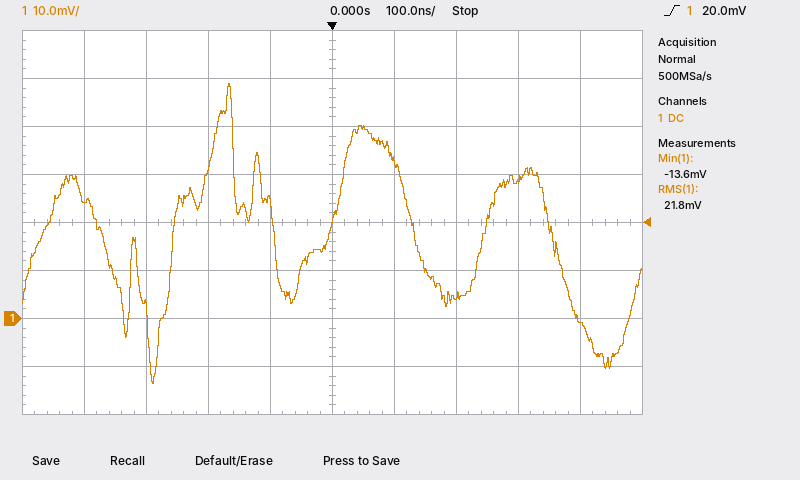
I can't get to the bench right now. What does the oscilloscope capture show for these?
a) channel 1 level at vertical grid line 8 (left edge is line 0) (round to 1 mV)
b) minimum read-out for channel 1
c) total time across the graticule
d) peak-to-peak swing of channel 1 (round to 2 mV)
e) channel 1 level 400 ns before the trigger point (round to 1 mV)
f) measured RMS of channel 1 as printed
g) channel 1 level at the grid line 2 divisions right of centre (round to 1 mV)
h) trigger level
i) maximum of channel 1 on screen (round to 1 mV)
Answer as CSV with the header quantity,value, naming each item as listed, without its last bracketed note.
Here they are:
quantity,value
channel 1 level at vertical grid line 8 (left edge is line 0),29 mV
minimum read-out for channel 1,-13.6 mV
total time across the graticule,1 µs
peak-to-peak swing of channel 1,62 mV
channel 1 level 400 ns before the trigger point,25 mV
measured RMS of channel 1 as printed,21.8 mV
channel 1 level at the grid line 2 divisions right of centre,5 mV
trigger level,20.0 mV
maximum of channel 1 on screen,49 mV
